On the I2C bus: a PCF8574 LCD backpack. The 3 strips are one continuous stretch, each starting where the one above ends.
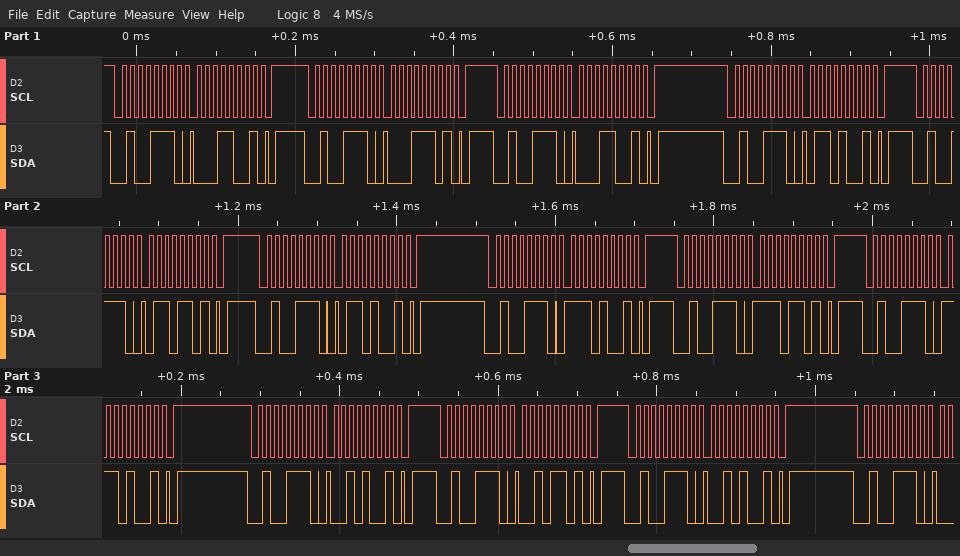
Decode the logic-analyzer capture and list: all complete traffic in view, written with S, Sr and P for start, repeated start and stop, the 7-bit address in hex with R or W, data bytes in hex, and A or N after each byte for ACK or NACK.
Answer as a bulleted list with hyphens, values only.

- S 27W A 19 A P S 27W A 1D A P S 27W A 19 A P S 27W A 69 A P S 27W A 6D A P S 27W A 69 A P S 27W A E9 A P S 27W A ED A P S 27W A E9 A P S 27W A 29 A P S 27W A 2D A P S 27W A 29 A P S 27W A
